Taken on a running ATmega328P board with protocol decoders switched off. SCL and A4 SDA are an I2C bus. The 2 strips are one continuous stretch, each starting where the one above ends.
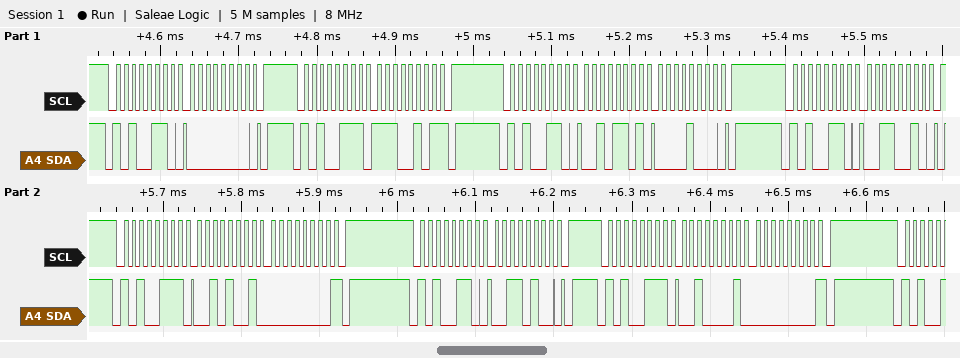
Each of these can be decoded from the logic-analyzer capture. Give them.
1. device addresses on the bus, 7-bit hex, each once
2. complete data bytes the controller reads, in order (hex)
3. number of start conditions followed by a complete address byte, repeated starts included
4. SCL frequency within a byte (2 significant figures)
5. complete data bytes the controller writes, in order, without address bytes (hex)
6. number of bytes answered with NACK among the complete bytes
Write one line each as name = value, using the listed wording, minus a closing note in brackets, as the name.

device addresses on the bus, 7-bit hex, each once = 0x53
complete data bytes the controller reads, in order = E5 29 00 21 00
number of start conditions followed by a complete address byte, repeated starts included = 7
SCL frequency within a byte = 100 kHz
complete data bytes the controller writes, in order, without address bytes = 00 2D 08 32 34
number of bytes answered with NACK among the complete bytes = 3
